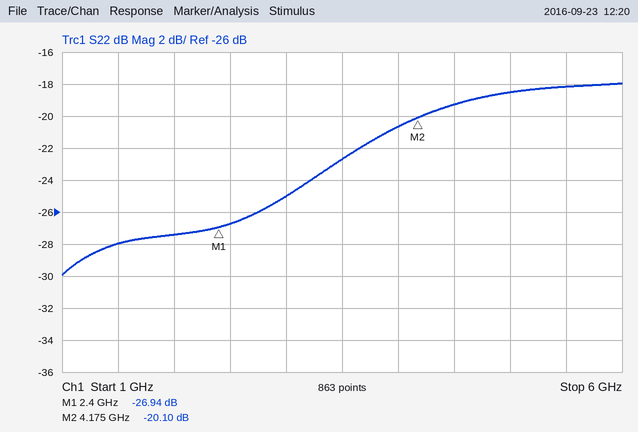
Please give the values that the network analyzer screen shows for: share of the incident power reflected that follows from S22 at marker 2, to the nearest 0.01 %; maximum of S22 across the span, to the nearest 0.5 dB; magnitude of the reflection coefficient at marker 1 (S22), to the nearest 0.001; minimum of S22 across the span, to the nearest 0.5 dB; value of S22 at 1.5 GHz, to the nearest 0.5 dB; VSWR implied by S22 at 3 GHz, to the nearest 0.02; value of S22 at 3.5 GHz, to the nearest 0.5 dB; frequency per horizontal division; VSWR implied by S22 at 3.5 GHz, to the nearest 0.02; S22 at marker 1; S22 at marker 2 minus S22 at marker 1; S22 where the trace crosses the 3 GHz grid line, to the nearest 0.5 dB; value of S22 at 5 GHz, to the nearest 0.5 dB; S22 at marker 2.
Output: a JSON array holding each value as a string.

["0.98 %", "-18.0 dB", "0.045", "-30.0 dB", "-28.0 dB", "1.12", "-22.5 dB", "500 MHz", "1.16", "-26.94 dB", "6.84 dB", "-25.0 dB", "-18.5 dB", "-20.10 dB"]
